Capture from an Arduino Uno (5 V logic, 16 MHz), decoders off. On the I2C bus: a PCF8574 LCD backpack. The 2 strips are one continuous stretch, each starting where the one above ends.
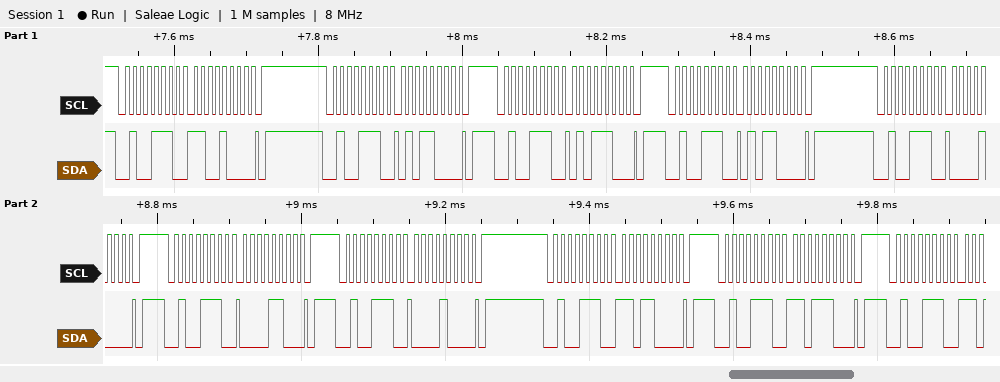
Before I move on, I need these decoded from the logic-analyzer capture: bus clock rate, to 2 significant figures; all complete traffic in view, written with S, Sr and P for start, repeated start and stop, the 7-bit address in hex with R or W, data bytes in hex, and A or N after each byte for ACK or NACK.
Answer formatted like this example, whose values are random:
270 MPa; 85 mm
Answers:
100 kHz; S 27W A C8 A P S 27W A 58 A P S 27W A 5C A P S 27W A 58 A P S 27W A 08 A P S 27W A 0C A P S 27W A 08 A P S 27W A D8 A P S 27W A DC A P S 27W A
